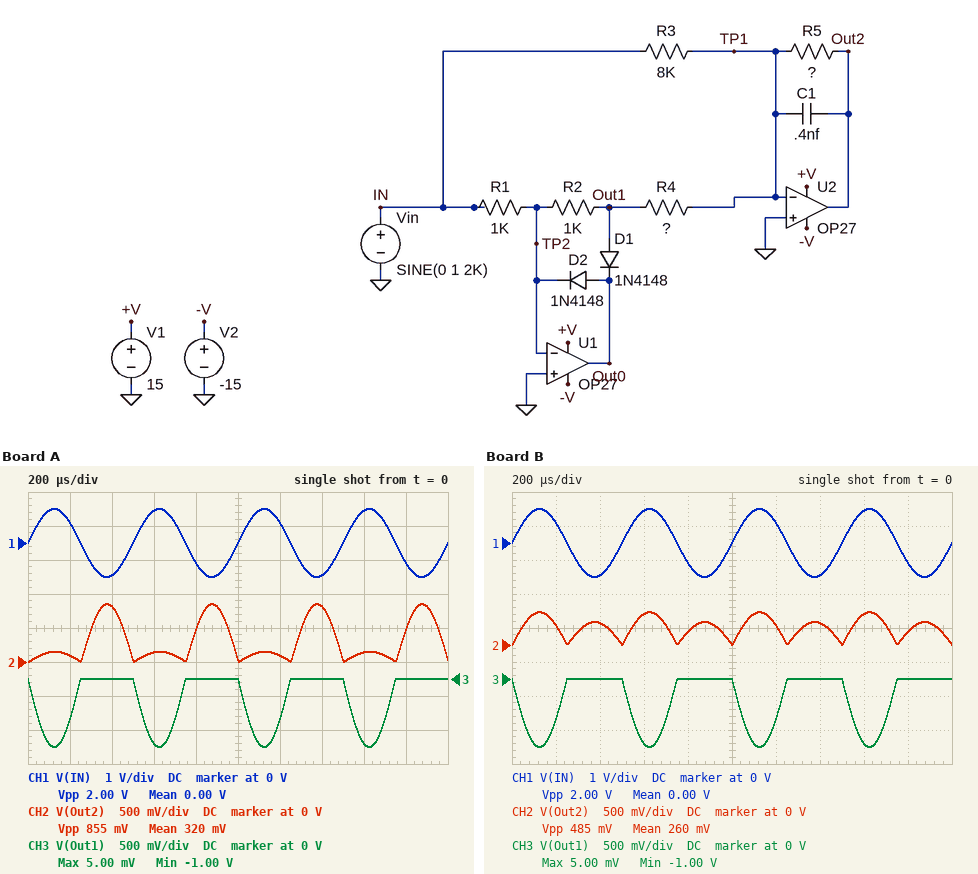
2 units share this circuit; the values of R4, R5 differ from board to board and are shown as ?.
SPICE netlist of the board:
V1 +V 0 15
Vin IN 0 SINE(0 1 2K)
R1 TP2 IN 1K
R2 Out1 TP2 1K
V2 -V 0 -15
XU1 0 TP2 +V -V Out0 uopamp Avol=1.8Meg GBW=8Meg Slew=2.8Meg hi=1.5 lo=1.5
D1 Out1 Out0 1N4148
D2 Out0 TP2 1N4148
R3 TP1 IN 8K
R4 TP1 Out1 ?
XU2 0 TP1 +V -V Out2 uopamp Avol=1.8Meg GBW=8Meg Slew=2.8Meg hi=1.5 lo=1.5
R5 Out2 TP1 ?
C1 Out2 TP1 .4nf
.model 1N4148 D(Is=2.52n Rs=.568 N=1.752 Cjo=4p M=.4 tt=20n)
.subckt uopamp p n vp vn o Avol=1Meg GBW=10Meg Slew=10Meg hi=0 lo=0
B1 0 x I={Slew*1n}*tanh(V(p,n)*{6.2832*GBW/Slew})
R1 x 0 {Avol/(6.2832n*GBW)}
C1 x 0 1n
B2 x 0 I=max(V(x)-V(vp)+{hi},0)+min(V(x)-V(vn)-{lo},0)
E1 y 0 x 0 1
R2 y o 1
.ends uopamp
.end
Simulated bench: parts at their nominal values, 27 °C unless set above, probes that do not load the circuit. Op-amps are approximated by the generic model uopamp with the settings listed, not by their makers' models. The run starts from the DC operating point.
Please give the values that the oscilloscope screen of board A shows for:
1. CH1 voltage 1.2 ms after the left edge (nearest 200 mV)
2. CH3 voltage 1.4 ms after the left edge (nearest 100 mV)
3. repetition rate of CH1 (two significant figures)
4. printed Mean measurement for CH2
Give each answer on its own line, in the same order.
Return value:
600 mV
0 V
2.0 kHz
320 mV
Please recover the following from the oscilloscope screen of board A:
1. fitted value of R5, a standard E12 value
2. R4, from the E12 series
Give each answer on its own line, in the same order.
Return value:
6.8 kΩ
6.8 kΩ
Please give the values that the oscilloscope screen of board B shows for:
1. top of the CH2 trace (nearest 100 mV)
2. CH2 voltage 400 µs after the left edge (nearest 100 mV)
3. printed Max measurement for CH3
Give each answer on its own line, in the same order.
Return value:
500 mV
300 mV
5.00 mV
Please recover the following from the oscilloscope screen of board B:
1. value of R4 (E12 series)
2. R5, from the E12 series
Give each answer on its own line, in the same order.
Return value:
3.3 kΩ
2.7 kΩ
